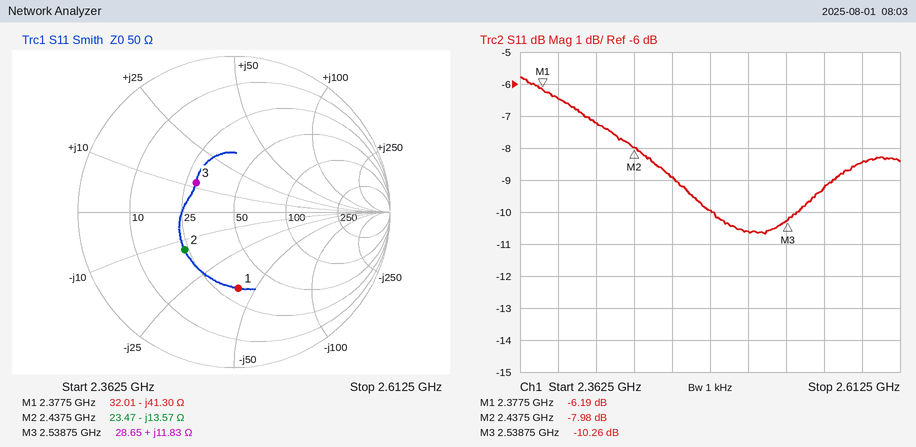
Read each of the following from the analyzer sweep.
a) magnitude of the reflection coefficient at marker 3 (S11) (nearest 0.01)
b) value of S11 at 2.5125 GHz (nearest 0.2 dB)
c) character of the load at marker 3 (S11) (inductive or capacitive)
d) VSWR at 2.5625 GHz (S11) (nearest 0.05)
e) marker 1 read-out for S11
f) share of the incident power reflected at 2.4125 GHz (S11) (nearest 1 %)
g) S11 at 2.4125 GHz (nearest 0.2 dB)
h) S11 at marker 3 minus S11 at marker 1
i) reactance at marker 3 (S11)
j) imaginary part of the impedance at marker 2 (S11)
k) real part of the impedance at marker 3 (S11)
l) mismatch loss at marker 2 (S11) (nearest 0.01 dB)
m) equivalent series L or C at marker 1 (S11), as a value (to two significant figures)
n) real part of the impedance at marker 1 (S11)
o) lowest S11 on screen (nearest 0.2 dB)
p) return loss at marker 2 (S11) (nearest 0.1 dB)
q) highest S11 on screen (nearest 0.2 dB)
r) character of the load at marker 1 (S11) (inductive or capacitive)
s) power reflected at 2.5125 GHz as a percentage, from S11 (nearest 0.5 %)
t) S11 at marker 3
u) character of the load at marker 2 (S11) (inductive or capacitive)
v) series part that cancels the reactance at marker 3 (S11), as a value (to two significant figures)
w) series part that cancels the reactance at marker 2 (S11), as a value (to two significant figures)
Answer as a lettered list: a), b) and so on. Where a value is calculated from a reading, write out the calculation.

a) 0.31
b) -10.6 dB
c) inductive
d) |Γ| = 10^(-9.2/20) = 0.3467; VSWR = (1 + 0.3467)/(1 − 0.3467) ≈ 2.06, so 2.05 to the nearest 0.05
e) -6.19 dB
f) 10^(-7.2/10) ≈ 19 %
g) -7.2 dB
h) -10.26 − (-6.19) = -4.07 dB
i) +11.83 Ω
j) -13.57 Ω
k) 28.65 Ω
l) −10 log10(1 − 10^(-7.98/10)) ≈ 0.75 dB
m) C = 1/(2π × 2.3775 GHz × 41.3 Ω) ≈ 1.6 pF
n) 32.01 Ω
o) -10.6 dB
p) 8.0 dB
q) -5.8 dB
r) capacitive
s) 10^(-10.6/10) ≈ 8.71 %, so 8.5 % to the nearest 0.5 %
t) -10.26 dB
u) capacitive
v) C = 1/(2π × 2.53875 GHz × 11.83 Ω) ≈ 5.3 pF
w) L = 13.57 Ω/(2π × 2.4375 GHz) ≈ 886 pH, so 890 pH to two significant figures
